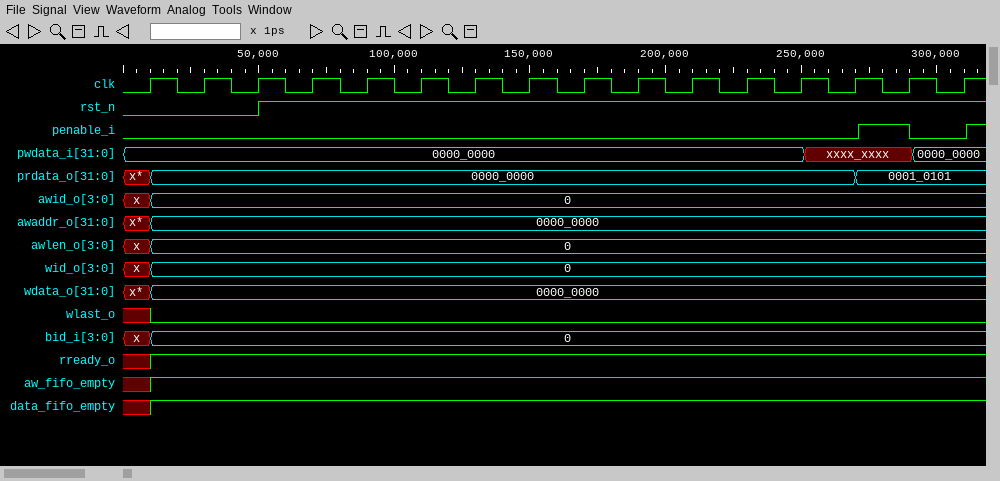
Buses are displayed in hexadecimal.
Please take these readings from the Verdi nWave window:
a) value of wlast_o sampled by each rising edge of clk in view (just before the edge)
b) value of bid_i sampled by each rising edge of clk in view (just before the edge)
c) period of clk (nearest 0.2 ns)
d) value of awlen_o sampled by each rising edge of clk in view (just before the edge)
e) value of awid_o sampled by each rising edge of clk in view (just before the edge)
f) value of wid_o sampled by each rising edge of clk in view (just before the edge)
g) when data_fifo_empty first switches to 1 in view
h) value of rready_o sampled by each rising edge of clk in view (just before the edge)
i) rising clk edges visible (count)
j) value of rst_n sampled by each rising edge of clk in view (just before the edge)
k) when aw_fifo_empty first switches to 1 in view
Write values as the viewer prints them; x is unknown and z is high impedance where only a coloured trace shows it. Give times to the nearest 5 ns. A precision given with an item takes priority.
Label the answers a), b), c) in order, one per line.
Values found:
a) x 0 0 0 0 0 0 0 0 0 0 0 0 0 0 0
b) x, 0, 0, 0, 0, 0, 0, 0, 0, 0, 0, 0, 0, 0, 0, 0
c) 20 ns
d) x, 0, 0, 0, 0, 0, 0, 0, 0, 0, 0, 0, 0, 0, 0, 0
e) x, 0, 0, 0, 0, 0, 0, 0, 0, 0, 0, 0, 0, 0, 0, 0
f) x, 0, 0, 0, 0, 0, 0, 0, 0, 0, 0, 0, 0, 0, 0, 0
g) 10 ns
h) x 1 1 1 1 1 1 1 1 1 1 1 1 1 1 1
i) 16
j) 0 0 0 1 1 1 1 1 1 1 1 1 1 1 1 1
k) 10 ns
